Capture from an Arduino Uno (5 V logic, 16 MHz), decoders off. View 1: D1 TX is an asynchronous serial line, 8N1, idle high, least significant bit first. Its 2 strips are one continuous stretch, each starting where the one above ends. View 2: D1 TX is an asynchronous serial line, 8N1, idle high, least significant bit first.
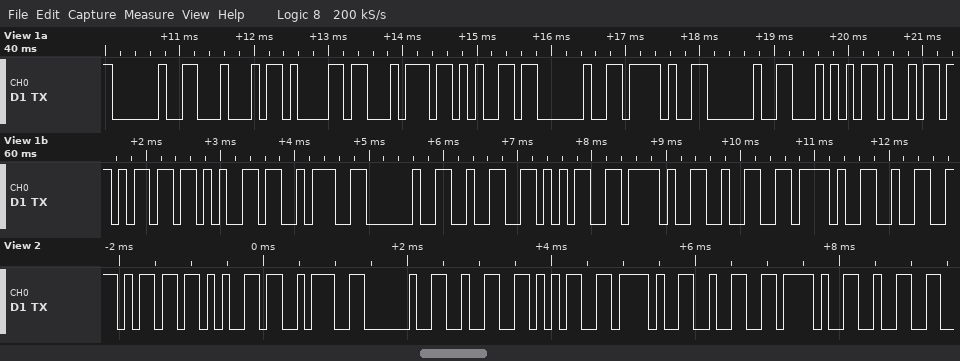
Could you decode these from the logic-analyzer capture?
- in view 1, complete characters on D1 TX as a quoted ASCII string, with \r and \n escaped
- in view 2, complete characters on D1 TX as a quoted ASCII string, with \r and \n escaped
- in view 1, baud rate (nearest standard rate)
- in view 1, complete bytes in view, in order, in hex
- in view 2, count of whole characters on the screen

" Date / Time: 25/2/2"
"me: 25/2/2"
9600 baud
20 44 61 74 65 20 2F 20 54 69 6D 65 3A 20 32 35 2F 32 2F 32
10
